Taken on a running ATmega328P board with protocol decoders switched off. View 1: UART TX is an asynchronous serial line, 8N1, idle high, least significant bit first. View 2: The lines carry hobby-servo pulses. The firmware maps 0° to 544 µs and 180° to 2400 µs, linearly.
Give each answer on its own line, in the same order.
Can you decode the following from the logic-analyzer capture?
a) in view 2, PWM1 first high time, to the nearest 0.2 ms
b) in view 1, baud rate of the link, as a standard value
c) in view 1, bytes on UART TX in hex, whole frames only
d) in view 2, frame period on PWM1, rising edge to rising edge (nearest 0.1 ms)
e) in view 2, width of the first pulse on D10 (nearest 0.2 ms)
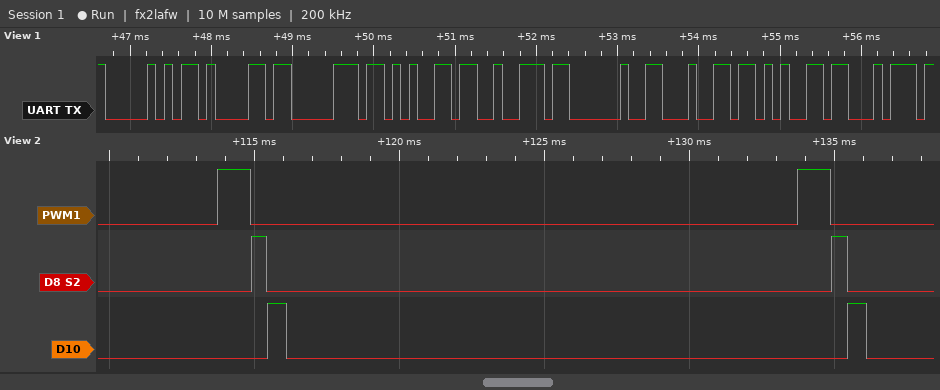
1.2 ms
9600 baud
50 61 70 65 72 20 64 65 74
20.0 ms
0.6 ms
